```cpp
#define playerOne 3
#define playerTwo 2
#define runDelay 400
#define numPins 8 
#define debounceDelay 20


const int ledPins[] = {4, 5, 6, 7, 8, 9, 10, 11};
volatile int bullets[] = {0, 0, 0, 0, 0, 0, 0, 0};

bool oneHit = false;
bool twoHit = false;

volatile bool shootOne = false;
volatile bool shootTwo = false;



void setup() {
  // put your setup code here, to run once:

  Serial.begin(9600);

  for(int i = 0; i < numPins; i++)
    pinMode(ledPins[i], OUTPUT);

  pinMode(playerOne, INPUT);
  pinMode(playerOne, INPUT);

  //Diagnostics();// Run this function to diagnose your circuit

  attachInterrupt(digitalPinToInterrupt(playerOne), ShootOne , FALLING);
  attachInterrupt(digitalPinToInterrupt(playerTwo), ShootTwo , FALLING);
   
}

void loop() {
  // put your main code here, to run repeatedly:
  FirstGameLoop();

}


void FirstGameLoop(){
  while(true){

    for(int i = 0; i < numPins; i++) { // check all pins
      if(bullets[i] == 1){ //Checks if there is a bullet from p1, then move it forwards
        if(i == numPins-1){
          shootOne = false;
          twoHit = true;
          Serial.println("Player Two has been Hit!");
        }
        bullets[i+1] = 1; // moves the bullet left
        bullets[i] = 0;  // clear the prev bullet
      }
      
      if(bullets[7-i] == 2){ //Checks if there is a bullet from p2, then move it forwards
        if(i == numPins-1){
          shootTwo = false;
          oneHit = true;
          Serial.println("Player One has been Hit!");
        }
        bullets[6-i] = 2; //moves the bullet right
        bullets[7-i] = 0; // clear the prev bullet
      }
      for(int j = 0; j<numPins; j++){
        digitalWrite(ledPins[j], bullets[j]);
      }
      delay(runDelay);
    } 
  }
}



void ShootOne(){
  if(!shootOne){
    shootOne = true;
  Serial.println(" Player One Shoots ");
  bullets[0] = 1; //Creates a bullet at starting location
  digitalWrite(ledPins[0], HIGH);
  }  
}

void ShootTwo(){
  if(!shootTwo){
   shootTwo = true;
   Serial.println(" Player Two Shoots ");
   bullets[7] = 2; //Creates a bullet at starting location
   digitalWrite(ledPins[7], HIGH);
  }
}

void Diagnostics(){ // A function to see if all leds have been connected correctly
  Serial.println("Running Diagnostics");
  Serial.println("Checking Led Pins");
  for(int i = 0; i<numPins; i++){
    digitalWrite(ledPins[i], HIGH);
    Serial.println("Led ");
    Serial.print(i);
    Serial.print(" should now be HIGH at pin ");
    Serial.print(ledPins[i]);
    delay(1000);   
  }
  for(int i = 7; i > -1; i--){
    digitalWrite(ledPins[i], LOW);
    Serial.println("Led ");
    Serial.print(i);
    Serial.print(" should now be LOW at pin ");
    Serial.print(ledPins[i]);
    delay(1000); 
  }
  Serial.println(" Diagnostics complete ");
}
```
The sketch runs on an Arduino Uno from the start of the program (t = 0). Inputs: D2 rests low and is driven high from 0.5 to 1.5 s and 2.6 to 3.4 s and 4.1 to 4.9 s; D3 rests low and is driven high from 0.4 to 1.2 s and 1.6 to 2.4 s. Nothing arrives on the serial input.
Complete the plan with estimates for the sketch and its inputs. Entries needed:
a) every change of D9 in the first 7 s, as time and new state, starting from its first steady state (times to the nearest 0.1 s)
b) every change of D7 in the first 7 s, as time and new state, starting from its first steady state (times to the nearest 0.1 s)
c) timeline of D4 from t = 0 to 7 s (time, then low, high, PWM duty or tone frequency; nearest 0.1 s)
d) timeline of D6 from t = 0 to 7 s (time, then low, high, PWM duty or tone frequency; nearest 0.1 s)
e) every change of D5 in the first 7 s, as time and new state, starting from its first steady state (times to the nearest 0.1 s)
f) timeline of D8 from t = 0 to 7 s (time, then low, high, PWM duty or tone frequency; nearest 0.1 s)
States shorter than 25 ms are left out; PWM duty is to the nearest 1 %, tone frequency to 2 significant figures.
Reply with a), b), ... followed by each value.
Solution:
a) 0 s low; 3.6 s high; 4 s low; 4.8 s high; 5.2 s low
b) 0 s low; 4 s high; 4.4 s low
c) 0 s low; 1.2 s high; 3.2 s low
d) 0 s low; 3.6 s high; 4 s low
e) 0 s low; 3.2 s high; 3.6 s low
f) 0 s low; 4 s high; 4.8 s low
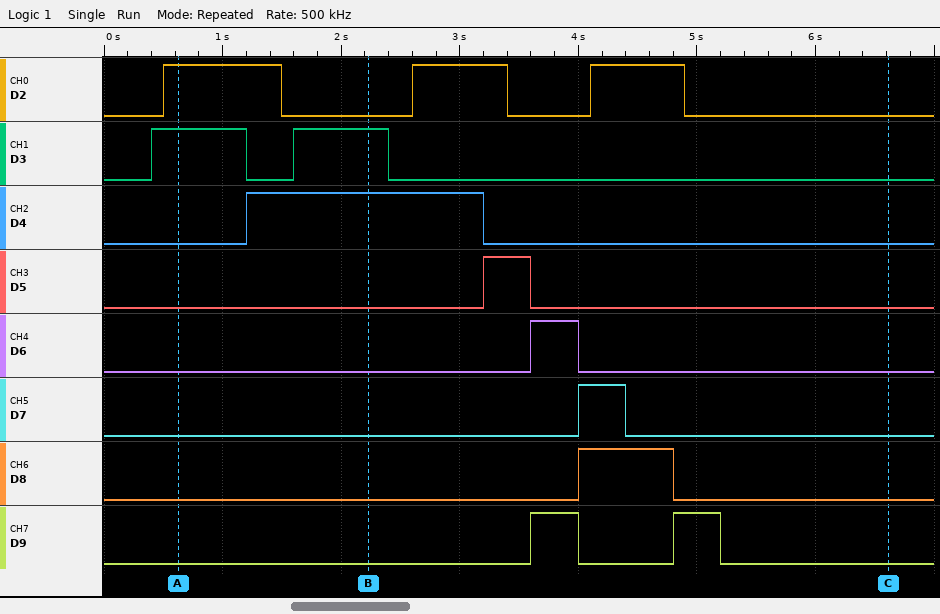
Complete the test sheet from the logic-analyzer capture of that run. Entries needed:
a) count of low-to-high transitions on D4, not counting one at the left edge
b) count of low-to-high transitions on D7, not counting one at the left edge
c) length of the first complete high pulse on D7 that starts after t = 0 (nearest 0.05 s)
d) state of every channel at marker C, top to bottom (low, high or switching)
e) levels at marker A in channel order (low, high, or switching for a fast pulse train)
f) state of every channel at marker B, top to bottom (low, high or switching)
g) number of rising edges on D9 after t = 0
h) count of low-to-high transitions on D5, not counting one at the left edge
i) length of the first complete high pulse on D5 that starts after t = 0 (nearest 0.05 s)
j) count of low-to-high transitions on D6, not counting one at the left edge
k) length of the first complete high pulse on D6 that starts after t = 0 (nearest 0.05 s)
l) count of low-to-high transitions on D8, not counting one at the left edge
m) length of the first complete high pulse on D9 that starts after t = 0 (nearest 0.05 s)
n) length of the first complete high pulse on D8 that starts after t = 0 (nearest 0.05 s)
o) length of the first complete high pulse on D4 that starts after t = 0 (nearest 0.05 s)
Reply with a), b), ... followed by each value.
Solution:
a) 1
b) 1
c) 0.40 s
d) D2 low, D3 low, D4 low, D5 low, D6 low, D7 low, D8 low, D9 low
e) D2 high, D3 high, D4 low, D5 low, D6 low, D7 low, D8 low, D9 low
f) D2 low, D3 high, D4 high, D5 low, D6 low, D7 low, D8 low, D9 low
g) 2
h) 1
i) 0.40 s
j) 1
k) 0.40 s
l) 1
m) 0.40 s
n) 0.80 s
o) 2.00 s
